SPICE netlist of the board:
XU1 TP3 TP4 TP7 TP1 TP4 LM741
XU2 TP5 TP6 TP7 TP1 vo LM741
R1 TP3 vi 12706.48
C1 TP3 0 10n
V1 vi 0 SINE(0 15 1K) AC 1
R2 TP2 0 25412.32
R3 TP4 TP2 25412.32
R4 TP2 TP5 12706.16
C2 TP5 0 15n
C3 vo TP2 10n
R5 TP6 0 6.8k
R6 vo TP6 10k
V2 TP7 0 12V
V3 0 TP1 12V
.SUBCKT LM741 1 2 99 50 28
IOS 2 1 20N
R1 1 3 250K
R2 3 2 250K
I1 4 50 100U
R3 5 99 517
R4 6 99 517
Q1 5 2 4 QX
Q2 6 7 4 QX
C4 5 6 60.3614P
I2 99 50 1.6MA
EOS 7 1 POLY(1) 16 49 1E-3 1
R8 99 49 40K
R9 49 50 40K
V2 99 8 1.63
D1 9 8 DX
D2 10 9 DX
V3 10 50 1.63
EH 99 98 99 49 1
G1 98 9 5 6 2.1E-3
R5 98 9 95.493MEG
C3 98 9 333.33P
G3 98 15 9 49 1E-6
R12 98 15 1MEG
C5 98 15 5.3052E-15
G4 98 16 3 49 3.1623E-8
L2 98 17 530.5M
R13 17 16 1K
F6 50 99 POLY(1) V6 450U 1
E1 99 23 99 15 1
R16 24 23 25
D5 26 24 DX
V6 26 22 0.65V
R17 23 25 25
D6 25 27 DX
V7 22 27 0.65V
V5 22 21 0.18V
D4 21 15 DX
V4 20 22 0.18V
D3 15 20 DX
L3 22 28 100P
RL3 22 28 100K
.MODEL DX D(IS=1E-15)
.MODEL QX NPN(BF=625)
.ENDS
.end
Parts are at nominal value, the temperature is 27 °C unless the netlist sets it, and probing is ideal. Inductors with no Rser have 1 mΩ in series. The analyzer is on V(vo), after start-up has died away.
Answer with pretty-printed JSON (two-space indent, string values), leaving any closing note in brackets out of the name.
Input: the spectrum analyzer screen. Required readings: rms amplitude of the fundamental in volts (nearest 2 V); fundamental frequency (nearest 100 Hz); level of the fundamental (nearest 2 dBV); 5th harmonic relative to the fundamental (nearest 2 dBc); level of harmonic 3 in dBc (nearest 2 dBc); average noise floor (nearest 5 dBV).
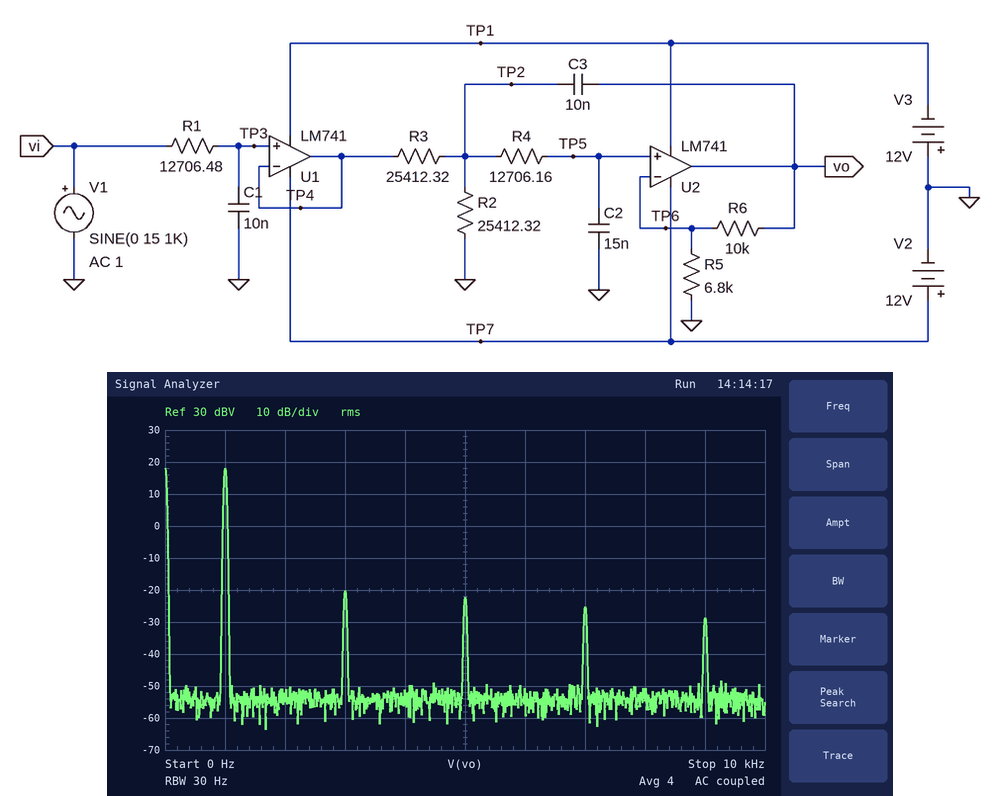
{
  "rms amplitude of the fundamental in volts": "8 V",
  "fundamental frequency": "1.0 kHz",
  "level of the fundamental": "18 dBV",
  "5th harmonic relative to the fundamental": "-40 dBc",
  "level of harmonic 3 in dBc": "-38 dBc",
  "average noise floor": "-55 dBV"
}
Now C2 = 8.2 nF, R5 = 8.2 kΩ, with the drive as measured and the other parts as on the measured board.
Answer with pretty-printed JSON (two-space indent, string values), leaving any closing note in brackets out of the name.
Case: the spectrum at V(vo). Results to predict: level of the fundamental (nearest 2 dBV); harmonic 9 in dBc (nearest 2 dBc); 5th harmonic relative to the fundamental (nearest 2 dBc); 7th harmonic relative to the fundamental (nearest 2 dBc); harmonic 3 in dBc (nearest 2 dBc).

{
  "level of the fundamental": "20 dBV",
  "harmonic 9 in dBc": "-38 dBc",
  "5th harmonic relative to the fundamental": "-30 dBc",
  "7th harmonic relative to the fundamental": "-32 dBc",
  "harmonic 3 in dBc": "-14 dBc"
}
